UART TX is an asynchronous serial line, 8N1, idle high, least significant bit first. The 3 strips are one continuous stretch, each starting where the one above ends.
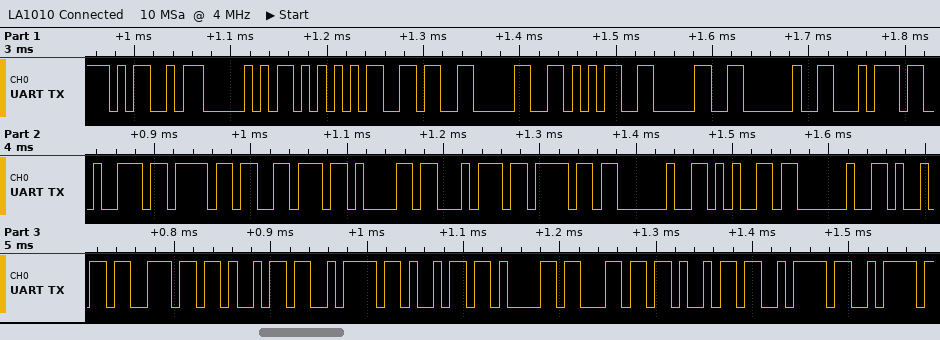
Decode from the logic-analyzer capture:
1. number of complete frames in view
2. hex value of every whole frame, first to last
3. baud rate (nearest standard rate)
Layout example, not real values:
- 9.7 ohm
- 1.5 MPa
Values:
- 28
- 4D 50 55 36 30 35 30 20 74 72 6F 76 61 74 6F 20 65 20 69 6E 69 7A 69 61 6C 69 7A 7A
- 115200 baud
